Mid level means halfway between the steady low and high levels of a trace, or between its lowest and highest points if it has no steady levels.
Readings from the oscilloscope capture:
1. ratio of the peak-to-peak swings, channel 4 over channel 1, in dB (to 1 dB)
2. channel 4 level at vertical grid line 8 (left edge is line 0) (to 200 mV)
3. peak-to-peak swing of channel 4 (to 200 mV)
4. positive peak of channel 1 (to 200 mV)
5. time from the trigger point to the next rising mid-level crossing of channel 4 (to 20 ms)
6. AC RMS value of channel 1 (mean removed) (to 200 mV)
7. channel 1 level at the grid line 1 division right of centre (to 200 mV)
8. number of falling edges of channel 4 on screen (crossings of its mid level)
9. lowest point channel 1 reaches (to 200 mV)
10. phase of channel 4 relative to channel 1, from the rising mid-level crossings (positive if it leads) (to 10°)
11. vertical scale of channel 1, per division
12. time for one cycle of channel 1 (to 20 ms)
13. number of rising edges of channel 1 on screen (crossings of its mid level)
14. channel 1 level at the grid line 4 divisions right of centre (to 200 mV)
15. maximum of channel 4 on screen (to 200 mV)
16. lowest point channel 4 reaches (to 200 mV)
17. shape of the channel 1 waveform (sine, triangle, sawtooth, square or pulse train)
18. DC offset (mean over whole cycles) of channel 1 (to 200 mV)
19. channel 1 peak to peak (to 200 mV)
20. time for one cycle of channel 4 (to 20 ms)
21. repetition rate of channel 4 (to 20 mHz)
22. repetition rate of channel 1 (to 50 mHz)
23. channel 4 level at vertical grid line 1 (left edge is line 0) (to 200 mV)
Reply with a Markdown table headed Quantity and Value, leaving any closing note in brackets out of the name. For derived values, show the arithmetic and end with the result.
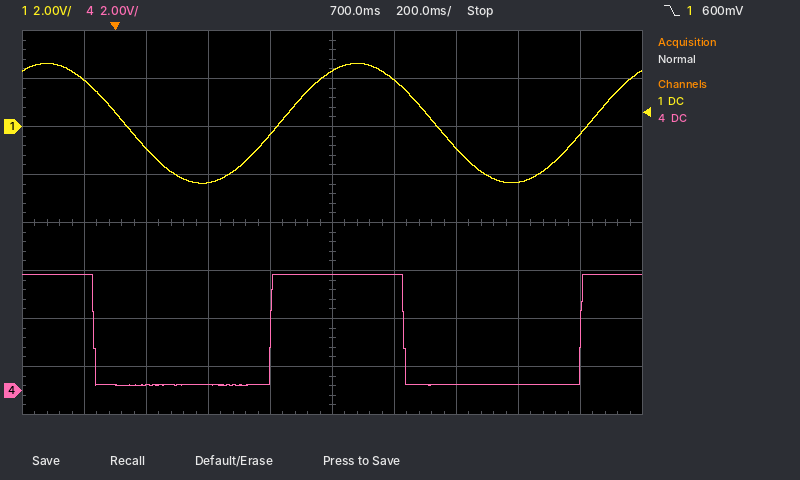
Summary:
| Quantity | Value |
|---|---|
| ratio of the peak-to-peak swings, channel 4 over channel 1, in dB | 20 log10(4.6 V / 5.0 V) ≈ -1 dB |
| channel 4 level at vertical grid line 8 (left edge is line 0) | 200 mV |
| peak-to-peak swing of channel 4 | 4.8 V − (200 mV) = 4.6 V |
| positive peak of channel 1 | 2.6 V |
| time from the trigger point to the next rising mid-level crossing of channel 4 | 500 ms |
| AC RMS value of channel 1 (mean removed) | 5.0 V / (2√2) ≈ 1.8 V |
| channel 1 level at the grid line 1 division right of centre | 2.0 V |
| number of falling edges of channel 4 on screen | 2 |
| lowest point channel 1 reaches | -2.4 V |
| phase of channel 4 relative to channel 1, from the rising mid-level crossings (positive if it leads) | +10° |
| vertical scale of channel 1, per division | 2 V |
| time for one cycle of channel 1 | 1.00 s |
| number of rising edges of channel 1 on screen | 2 |
| channel 1 level at the grid line 4 divisions right of centre | -400 mV |
| maximum of channel 4 on screen | 4.8 V |
| lowest point channel 4 reaches | 200 mV |
| shape of the channel 1 waveform | sine |
| DC offset (mean over whole cycles) of channel 1 | (2.6 V + (-2.4 V)) / 2 ≈ 100 mV, so 200 mV to the nearest 200 mV |
| channel 1 peak to peak | 2.6 V − (-2.4 V) = 5.0 V |
| time for one cycle of channel 4 | 1.00 s |
| repetition rate of channel 4 | 1 / 1.00 s ≈ 1.00 Hz |
| repetition rate of channel 1 | 1 / 1.00 s ≈ 1.00 Hz |
| channel 4 level at vertical grid line 1 (left edge is line 0) | 4.8 V |
